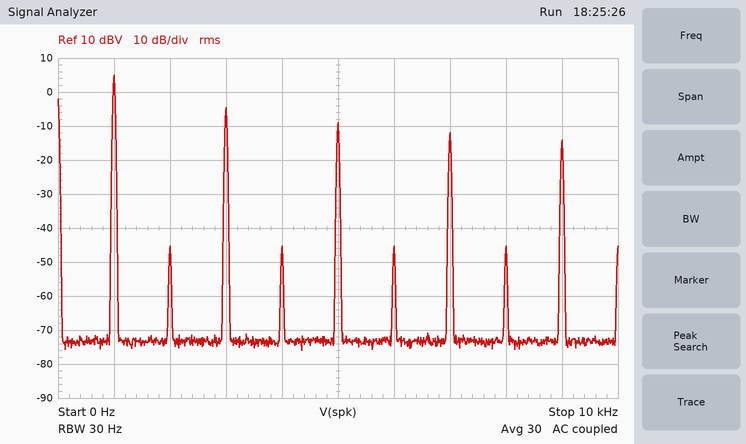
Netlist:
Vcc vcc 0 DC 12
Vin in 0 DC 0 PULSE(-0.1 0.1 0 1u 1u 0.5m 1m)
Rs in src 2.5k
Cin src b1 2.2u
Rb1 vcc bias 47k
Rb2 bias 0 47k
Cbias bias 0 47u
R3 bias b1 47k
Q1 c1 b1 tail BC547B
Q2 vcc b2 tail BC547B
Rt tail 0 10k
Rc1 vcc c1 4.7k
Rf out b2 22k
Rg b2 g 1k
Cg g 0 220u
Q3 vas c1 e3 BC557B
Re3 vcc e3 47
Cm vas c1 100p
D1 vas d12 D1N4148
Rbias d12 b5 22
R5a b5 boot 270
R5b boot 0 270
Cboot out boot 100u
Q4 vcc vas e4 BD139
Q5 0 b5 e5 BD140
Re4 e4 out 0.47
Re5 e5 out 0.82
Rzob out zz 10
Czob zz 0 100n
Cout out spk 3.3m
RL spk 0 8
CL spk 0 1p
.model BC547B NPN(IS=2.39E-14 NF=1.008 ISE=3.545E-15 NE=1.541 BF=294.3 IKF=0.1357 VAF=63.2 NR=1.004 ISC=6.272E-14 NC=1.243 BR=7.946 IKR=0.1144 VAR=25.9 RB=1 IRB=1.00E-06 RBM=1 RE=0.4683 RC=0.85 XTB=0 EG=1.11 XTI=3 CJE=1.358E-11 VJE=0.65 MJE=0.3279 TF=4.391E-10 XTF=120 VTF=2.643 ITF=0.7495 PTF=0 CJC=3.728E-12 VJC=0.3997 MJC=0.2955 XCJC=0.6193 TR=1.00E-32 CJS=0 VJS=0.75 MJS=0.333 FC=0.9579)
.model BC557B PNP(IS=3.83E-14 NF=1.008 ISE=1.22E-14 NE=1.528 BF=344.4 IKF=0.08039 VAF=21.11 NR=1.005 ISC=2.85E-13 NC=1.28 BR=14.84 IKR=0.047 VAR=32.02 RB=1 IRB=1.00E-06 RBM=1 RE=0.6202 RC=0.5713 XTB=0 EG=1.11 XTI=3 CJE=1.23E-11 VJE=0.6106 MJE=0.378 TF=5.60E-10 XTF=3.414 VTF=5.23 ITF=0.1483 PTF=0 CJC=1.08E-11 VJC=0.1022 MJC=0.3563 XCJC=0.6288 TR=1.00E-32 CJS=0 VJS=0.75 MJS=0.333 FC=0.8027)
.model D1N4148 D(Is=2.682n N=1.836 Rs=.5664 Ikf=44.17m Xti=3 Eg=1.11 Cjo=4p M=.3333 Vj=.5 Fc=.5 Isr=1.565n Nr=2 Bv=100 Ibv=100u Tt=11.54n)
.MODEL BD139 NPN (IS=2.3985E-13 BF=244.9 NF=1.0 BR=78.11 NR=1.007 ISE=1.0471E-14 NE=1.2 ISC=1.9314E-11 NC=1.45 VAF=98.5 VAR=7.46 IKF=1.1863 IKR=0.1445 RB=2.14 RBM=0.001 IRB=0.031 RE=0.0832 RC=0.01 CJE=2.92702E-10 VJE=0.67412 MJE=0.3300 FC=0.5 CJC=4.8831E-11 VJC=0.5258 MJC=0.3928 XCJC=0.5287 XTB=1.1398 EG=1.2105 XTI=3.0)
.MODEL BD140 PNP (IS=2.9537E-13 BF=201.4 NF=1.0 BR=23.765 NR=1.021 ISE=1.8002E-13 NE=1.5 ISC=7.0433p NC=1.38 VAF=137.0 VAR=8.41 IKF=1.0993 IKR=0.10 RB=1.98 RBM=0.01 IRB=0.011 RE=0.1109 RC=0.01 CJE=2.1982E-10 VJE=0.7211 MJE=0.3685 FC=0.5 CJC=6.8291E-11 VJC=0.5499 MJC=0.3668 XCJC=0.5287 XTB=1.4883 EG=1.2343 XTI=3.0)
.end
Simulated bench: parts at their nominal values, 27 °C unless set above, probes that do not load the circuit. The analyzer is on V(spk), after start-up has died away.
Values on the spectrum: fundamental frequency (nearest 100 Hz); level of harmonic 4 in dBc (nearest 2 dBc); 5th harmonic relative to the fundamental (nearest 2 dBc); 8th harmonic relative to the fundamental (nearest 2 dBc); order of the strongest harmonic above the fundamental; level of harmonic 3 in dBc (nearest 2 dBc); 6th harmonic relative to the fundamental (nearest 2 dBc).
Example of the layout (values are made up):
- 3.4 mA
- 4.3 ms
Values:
- 1.0 kHz
- -50 dBc
- -14 dBc
- -50 dBc
- 3
- -10 dBc
- -50 dBc
